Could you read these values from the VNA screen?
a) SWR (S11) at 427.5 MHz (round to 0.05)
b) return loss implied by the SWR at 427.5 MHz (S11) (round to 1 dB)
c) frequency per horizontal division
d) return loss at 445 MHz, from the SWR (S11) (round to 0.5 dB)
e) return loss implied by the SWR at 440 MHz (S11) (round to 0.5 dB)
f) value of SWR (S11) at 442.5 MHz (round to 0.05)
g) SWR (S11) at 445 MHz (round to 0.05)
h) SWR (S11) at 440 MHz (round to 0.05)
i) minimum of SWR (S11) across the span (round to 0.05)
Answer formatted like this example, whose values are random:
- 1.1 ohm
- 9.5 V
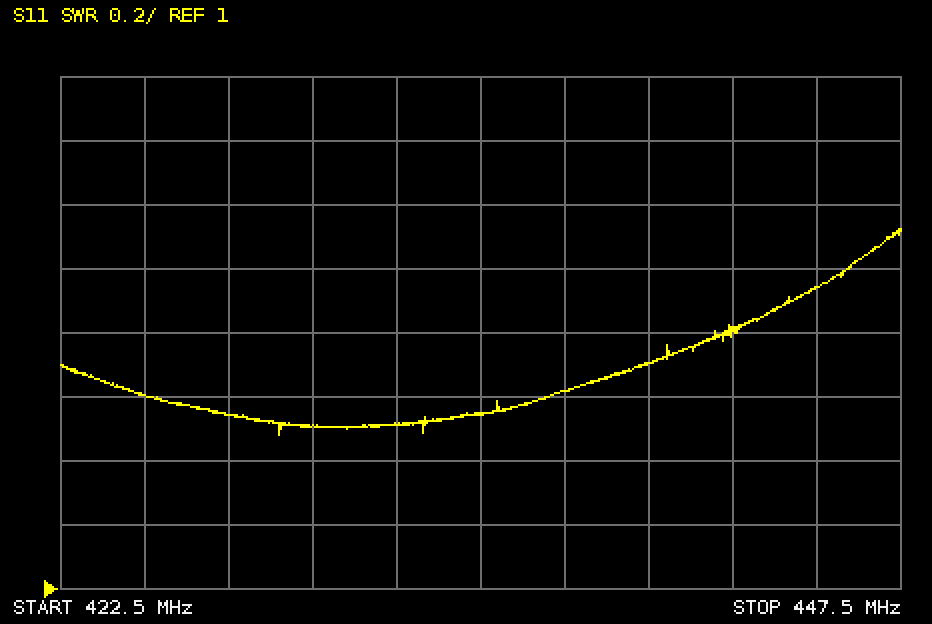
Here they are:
- 1.55
- 13 dB
- 2.5 MHz
- 10.0 dB
- 11.5 dB
- 1.80
- 1.95
- 1.70
- 1.50
